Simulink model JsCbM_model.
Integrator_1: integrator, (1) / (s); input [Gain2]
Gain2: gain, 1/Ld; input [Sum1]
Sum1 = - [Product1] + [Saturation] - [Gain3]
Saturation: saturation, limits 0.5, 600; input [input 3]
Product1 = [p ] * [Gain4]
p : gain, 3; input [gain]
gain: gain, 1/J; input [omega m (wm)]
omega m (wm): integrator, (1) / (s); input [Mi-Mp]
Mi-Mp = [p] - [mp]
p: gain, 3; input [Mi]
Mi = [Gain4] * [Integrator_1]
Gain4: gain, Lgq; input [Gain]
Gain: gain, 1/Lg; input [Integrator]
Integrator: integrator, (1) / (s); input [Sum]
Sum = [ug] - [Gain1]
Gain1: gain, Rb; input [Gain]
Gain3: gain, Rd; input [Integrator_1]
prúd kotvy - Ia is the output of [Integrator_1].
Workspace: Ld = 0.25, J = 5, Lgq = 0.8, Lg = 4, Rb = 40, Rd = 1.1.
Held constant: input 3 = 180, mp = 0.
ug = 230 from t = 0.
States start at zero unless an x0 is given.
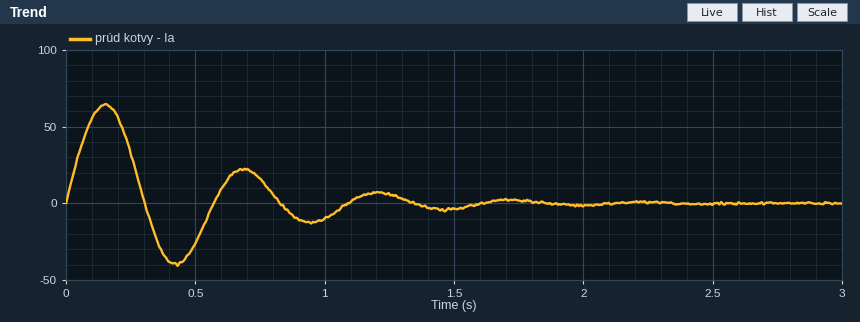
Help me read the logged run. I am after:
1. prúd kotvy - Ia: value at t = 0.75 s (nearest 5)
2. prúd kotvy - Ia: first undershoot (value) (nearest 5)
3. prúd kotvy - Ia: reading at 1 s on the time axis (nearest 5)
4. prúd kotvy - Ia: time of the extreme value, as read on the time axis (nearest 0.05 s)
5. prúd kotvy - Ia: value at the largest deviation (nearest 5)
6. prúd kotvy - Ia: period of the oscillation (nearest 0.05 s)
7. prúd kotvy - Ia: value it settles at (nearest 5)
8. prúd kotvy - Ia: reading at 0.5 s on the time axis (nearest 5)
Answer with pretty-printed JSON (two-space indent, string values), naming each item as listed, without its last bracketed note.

{
  "prúd kotvy - Ia: value at t = 0.75 s": "15",
  "prúd kotvy - Ia: first undershoot (value)": "-40",
  "prúd kotvy - Ia: reading at 1 s on the time axis": "-10",
  "prúd kotvy - Ia: time of the extreme value, as read on the time axis": "0.15 s",
  "prúd kotvy - Ia: value at the largest deviation": "65",
  "prúd kotvy - Ia: period of the oscillation": "0.55 s",
  "prúd kotvy - Ia: value it settles at": "0",
  "prúd kotvy - Ia: reading at 0.5 s on the time axis": "-25"
}
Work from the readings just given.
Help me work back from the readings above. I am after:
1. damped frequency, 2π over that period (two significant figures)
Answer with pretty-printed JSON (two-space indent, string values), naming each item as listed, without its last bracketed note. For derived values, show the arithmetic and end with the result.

{
  "damped frequency, 2π over that period": "2π / 0.55 = 11 rad/s"
}
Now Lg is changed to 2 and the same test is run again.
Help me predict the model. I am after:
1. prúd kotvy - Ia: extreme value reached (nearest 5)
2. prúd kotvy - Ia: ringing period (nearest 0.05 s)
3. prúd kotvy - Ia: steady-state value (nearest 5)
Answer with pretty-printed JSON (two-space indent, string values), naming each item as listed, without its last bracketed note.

{
  "prúd kotvy - Ia: extreme value reached": "55",
  "prúd kotvy - Ia: ringing period": "0.50 s",
  "prúd kotvy - Ia: steady-state value": "0"
}
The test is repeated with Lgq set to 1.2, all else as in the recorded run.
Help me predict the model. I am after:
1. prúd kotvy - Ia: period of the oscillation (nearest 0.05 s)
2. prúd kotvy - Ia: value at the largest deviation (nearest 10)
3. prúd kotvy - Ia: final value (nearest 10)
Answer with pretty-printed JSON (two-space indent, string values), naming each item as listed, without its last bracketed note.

{
  "prúd kotvy - Ia: period of the oscillation": "0.35 s",
  "prúd kotvy - Ia: value at the largest deviation": "50",
  "prúd kotvy - Ia: final value": "0"
}
